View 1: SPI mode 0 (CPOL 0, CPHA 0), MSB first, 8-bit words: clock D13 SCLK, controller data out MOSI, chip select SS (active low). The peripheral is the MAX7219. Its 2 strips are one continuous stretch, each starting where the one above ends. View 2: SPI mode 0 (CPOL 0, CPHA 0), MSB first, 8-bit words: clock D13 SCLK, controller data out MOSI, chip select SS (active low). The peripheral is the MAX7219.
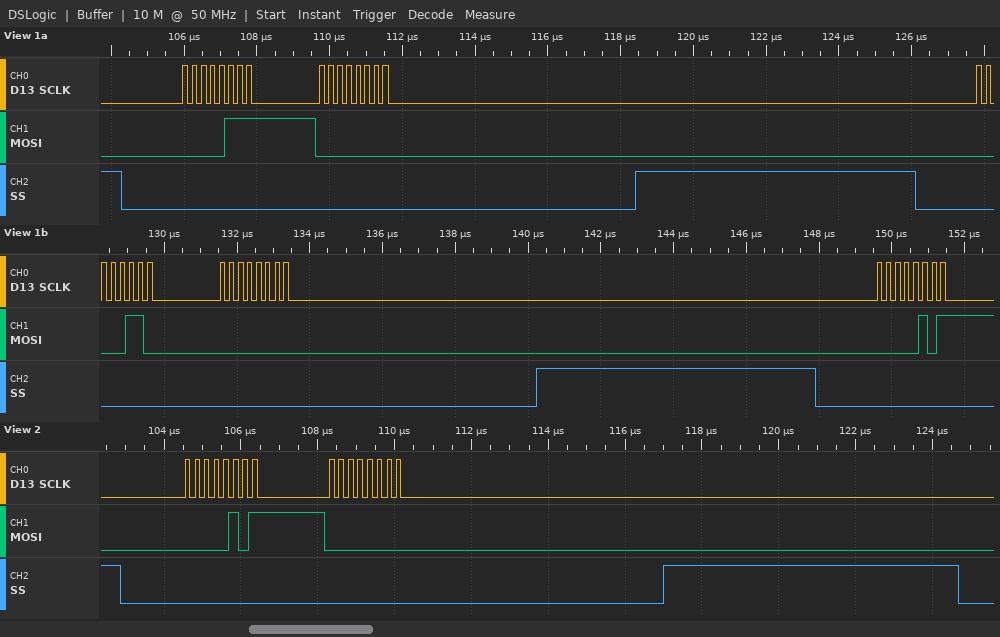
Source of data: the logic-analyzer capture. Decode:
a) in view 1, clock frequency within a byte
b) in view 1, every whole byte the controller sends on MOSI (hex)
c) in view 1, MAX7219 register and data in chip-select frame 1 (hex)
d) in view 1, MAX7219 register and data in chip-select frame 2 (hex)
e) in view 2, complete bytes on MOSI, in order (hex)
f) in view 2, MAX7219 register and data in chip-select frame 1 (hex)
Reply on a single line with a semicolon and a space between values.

4 MHz; 0x07 0x00 0x06 0x00 0x05; register 0x7, data 0x00; register 0x6, data 0x00; 05 00; register 0x5, data 0x00
